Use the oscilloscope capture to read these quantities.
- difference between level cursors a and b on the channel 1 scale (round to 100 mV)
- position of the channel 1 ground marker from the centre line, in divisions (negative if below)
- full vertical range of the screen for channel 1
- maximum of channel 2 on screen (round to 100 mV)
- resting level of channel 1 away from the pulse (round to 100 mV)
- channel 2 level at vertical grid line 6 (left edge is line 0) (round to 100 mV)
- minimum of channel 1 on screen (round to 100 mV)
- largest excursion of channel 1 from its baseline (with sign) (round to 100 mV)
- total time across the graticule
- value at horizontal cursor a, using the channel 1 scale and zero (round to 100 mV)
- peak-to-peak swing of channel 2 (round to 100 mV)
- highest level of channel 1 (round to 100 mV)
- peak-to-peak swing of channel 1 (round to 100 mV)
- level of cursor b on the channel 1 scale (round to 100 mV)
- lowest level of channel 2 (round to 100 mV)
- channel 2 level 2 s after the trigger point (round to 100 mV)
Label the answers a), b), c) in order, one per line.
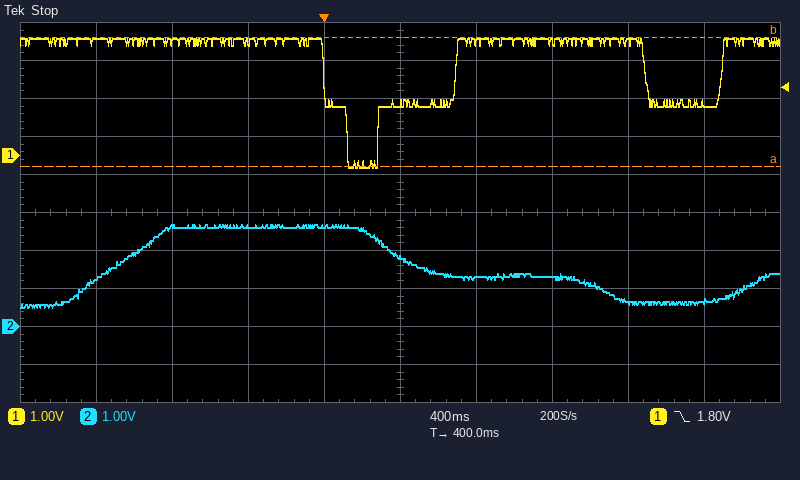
a) 3.4 V
b) +1.5 div
c) 10 V
d) 2.7 V
e) 3.1 V
f) 1.3 V
g) -300 mV
h) -3.4 V
i) 4 s
j) -300 mV
k) 2.2 V
l) 3.1 V
m) 3.4 V
n) 3.1 V
o) 500 mV
p) 700 mV
